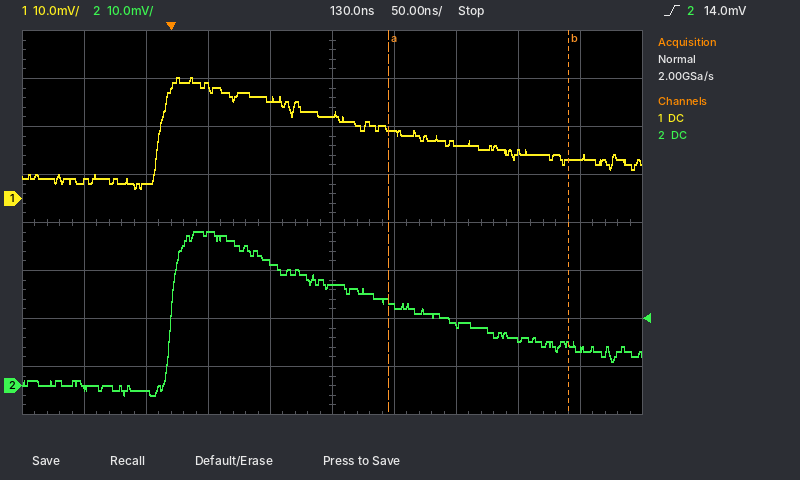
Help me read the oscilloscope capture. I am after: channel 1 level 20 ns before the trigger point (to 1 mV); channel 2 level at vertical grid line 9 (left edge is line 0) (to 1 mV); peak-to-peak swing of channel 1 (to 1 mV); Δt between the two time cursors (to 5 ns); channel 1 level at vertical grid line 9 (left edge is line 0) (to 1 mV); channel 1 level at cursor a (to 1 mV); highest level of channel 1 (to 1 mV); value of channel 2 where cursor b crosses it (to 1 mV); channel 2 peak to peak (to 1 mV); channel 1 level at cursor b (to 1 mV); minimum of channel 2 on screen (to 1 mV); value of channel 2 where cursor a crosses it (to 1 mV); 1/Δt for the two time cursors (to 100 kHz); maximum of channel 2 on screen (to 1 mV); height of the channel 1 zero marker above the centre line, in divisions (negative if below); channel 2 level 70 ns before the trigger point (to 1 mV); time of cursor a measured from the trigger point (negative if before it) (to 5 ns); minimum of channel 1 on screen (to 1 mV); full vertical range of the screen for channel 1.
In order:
3 mV
8 mV
23 mV
145 ns
8 mV
15 mV
25 mV
9 mV
34 mV
8 mV
-2 mV
18 mV
6.9 MHz
32 mV
+0.5 div
0 mV
+175 ns
2 mV
80 mV
